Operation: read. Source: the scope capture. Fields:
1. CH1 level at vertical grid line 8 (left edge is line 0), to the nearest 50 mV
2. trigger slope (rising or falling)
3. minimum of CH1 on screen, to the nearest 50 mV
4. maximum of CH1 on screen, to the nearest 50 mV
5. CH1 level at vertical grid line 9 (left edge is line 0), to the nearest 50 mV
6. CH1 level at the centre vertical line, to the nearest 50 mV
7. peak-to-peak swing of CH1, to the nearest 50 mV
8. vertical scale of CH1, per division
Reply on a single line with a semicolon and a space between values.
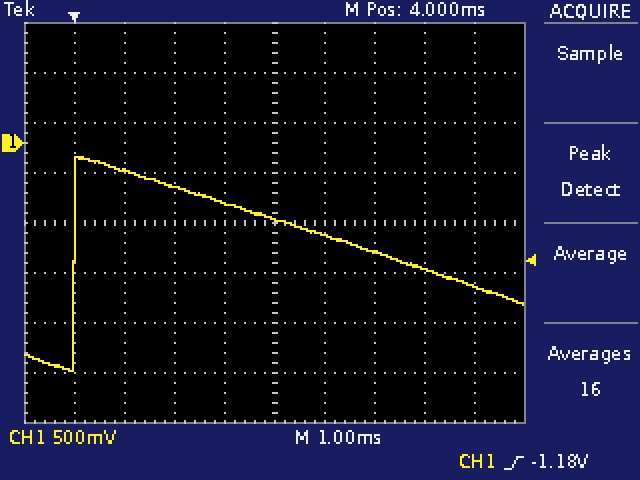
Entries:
-1.25 V; rising; -2.30 V; -150 mV; -1.45 V; -750 mV; 2.15 V; 500 mV
